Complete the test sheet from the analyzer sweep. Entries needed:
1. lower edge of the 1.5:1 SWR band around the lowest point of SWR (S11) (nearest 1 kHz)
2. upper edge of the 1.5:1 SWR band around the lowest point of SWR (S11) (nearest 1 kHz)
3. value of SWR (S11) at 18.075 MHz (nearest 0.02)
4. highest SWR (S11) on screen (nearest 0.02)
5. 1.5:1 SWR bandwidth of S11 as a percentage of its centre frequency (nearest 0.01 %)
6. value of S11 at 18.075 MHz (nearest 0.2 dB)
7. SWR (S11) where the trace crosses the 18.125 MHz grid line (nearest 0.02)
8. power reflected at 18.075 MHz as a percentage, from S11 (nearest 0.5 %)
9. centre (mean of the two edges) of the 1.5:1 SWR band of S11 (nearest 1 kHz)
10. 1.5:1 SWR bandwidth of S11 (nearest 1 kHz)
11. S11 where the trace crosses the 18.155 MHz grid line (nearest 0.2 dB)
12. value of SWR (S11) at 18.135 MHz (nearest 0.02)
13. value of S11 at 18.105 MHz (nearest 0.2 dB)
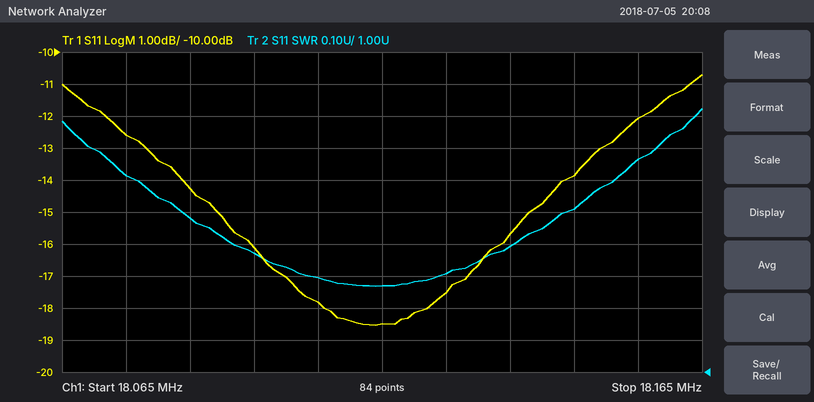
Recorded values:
18.084 MHz
18.144 MHz
1.62
1.82
0.33 %
-12.6 dB
1.30
5.5 %
18.114 MHz
60 kHz
-12.0 dB
1.40
-17.8 dB
